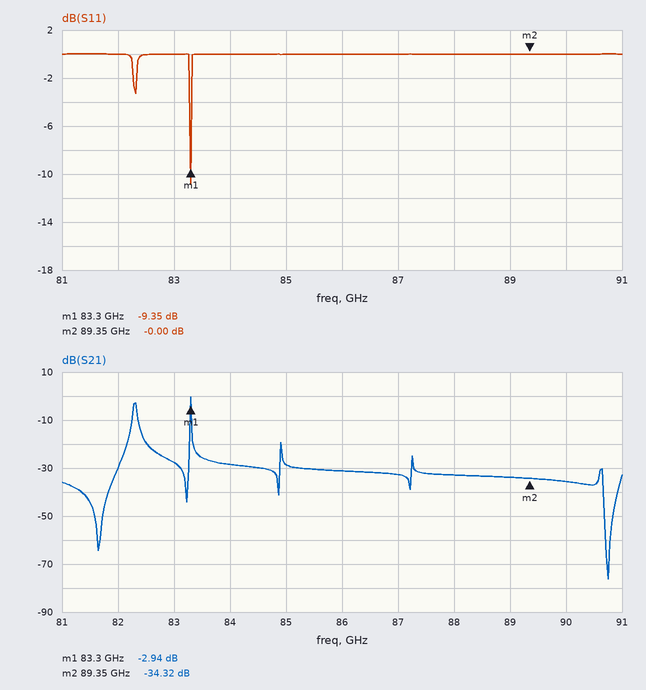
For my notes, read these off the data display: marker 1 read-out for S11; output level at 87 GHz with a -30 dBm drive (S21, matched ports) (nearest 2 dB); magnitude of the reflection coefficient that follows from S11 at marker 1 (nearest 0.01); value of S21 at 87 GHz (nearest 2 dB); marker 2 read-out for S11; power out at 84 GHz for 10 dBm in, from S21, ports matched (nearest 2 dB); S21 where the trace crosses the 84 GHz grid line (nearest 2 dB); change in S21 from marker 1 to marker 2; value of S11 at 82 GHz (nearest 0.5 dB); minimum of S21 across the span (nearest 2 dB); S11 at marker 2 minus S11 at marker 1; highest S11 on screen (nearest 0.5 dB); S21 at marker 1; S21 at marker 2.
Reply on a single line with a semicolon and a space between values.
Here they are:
-9.35 dB; -62 dBm; 0.34; -32 dB; -0.00 dB; -18 dBm; -28 dB; -31.38 dB; 0.0 dB; -76 dB; 9.35 dB; 0.0 dB; -2.94 dB; -34.32 dB
